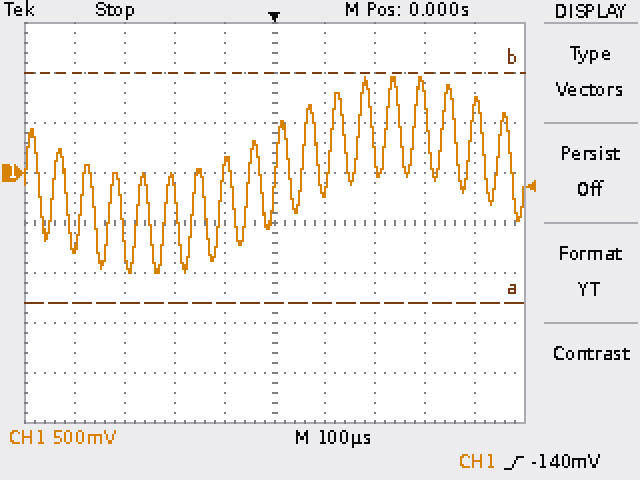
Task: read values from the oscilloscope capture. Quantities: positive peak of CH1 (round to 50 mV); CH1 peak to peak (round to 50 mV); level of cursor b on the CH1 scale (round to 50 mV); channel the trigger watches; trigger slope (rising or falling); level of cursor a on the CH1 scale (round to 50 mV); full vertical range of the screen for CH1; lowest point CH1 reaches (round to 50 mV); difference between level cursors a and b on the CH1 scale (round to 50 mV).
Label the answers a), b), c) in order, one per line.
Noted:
a) 950 mV
b) 1.95 V
c) 1.00 V
d) CH1
e) rising
f) -1.30 V
g) 4 V
h) -1.00 V
i) 2.30 V
